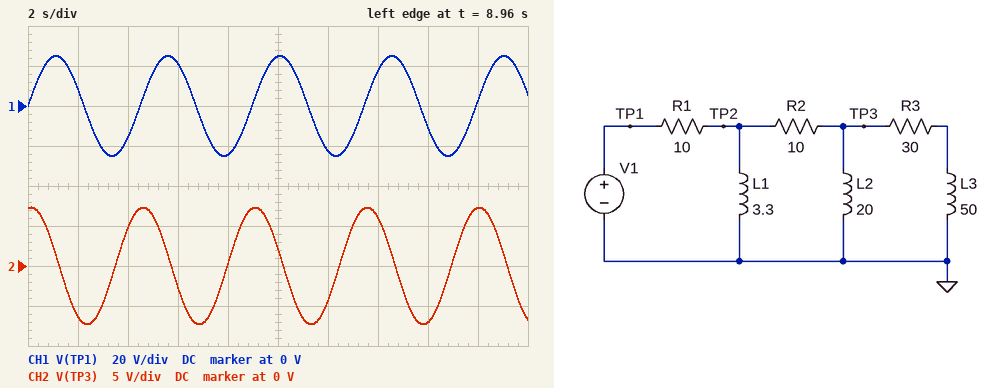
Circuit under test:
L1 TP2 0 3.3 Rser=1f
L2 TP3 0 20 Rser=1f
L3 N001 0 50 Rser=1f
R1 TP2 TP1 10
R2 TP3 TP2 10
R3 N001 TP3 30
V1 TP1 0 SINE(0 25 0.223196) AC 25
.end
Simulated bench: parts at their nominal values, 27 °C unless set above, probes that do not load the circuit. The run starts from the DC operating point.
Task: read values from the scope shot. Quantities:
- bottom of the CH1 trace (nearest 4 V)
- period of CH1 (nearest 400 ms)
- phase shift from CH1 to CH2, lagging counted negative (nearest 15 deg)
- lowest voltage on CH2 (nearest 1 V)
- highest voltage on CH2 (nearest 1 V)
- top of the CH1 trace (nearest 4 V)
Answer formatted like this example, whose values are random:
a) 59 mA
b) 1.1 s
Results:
a) -24 V
b) 4.4 s
c) 75 deg
d) -7 V
e) 7 V
f) 24 V
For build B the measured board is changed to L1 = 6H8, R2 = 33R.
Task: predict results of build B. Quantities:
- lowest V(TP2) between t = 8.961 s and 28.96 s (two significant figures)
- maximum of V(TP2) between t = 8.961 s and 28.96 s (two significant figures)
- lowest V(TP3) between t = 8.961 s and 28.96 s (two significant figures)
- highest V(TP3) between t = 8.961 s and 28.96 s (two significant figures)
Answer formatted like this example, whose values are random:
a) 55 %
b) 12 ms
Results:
a) -14 V
b) 14 V
c) -7.2 V
d) 7.2 V
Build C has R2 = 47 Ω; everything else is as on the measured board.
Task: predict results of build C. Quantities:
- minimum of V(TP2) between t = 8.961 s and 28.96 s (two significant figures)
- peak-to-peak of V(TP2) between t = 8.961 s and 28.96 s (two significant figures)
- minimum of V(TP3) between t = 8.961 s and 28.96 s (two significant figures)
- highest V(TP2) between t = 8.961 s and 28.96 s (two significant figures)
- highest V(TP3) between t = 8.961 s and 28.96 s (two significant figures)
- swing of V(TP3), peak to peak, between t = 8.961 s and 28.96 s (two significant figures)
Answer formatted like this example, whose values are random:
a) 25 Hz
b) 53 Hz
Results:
a) -9.3 V
b) 19 V
c) -3.6 V
d) 9.3 V
e) 3.6 V
f) 7.2 V
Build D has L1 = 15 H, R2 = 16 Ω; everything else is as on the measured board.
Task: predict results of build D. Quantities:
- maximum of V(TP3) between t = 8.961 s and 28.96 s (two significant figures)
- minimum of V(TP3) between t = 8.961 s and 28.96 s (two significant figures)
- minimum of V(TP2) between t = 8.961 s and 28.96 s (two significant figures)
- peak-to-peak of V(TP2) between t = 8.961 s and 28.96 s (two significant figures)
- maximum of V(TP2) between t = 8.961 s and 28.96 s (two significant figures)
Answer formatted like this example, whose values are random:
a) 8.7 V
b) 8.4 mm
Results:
a) 13 V
b) -13 V
c) -17 V
d) 34 V
e) 17 V
